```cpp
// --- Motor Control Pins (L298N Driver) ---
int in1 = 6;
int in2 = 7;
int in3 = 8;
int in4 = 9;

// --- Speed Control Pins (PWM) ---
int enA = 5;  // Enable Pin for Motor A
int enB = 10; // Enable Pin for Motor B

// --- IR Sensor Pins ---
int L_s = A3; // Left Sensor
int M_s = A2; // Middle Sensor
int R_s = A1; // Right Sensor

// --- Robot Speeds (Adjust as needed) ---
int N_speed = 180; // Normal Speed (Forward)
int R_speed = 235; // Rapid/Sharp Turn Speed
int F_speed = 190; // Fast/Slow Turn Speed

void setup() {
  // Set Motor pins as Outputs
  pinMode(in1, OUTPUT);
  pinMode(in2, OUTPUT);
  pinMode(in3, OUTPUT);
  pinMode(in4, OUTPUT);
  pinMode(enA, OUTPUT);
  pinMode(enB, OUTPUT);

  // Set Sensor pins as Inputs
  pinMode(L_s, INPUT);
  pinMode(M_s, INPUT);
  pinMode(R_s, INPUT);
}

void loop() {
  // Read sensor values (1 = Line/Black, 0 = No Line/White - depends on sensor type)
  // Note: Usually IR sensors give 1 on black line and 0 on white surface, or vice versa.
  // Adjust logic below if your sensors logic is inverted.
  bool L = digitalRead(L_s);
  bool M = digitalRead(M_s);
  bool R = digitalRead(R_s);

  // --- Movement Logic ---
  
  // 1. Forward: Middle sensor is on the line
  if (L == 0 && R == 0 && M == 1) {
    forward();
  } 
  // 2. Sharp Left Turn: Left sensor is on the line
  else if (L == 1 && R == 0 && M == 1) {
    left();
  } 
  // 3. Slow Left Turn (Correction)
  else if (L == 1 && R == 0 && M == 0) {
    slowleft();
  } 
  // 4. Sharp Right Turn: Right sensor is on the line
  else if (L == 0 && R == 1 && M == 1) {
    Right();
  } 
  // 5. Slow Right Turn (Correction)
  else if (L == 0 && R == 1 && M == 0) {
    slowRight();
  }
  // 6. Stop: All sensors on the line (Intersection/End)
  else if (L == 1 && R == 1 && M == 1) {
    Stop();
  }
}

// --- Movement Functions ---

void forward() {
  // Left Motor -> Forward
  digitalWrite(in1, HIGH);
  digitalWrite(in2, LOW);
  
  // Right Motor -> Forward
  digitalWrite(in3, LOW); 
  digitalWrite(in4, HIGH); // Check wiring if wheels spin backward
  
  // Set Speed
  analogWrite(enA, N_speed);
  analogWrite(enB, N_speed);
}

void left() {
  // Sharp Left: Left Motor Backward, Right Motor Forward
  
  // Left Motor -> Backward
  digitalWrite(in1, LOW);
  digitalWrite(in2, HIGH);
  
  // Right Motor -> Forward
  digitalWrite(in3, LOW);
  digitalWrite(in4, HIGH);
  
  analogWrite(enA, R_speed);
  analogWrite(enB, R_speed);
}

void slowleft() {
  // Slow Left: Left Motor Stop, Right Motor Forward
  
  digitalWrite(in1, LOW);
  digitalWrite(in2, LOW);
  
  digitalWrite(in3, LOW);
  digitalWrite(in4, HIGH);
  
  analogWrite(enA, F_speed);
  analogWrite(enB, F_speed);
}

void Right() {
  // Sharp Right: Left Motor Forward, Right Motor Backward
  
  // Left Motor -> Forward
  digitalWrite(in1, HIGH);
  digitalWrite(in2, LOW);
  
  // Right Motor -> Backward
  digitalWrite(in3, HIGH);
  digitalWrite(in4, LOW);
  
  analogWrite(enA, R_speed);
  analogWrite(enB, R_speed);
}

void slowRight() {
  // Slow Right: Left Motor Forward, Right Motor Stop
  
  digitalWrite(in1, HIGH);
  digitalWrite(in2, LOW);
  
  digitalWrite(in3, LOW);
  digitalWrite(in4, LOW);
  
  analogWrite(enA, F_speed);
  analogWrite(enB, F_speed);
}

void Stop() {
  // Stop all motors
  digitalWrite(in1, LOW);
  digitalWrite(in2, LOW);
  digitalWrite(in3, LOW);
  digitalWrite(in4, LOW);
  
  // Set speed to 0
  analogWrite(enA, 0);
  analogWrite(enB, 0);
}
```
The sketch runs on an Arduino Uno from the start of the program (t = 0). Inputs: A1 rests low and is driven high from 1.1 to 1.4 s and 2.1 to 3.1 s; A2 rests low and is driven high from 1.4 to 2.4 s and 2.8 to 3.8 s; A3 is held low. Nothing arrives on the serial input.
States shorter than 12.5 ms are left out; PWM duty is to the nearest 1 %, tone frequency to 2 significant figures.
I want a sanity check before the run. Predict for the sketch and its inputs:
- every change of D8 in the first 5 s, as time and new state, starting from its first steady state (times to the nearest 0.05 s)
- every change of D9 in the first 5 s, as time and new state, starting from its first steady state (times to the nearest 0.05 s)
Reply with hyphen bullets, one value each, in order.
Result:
- 0 s low; 2.1 s high; 2.4 s low; 2.8 s high; 3.1 s low
- 0 s low; 1.4 s high; 2.1 s low; 3.1 s high
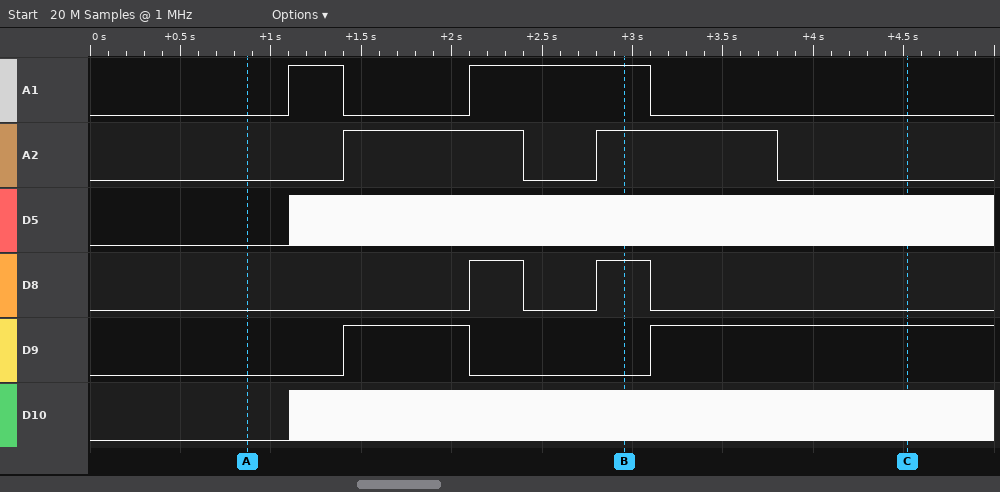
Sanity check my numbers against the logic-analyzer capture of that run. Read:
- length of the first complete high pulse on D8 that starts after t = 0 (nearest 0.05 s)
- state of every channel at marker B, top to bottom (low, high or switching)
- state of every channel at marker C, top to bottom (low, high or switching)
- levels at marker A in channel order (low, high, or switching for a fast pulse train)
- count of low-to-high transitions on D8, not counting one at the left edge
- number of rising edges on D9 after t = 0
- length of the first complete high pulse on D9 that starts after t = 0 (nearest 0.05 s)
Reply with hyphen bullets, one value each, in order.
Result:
- 0.30 s
- A1 high, A2 high, D5 switching, D8 high, D9 low, D10 switching
- A1 low, A2 low, D5 switching, D8 low, D9 high, D10 switching
- A1 low, A2 low, D5 low, D8 low, D9 low, D10 low
- 2
- 2
- 0.70 s
